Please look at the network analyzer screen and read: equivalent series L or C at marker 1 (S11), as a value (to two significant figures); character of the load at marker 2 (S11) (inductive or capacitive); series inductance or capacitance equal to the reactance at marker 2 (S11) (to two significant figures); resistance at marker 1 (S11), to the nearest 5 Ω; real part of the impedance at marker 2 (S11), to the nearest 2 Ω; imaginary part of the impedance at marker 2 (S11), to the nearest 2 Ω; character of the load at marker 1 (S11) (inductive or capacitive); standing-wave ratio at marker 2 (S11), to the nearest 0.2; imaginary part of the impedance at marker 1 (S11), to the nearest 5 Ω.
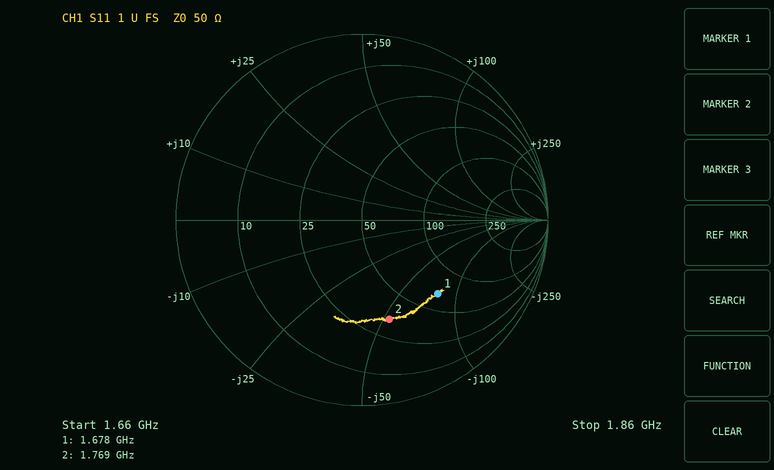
1.2 pF
capacitive
1.7 pF
65 Ω
34 Ω
-52 Ω
capacitive
3.4
-80 Ω
